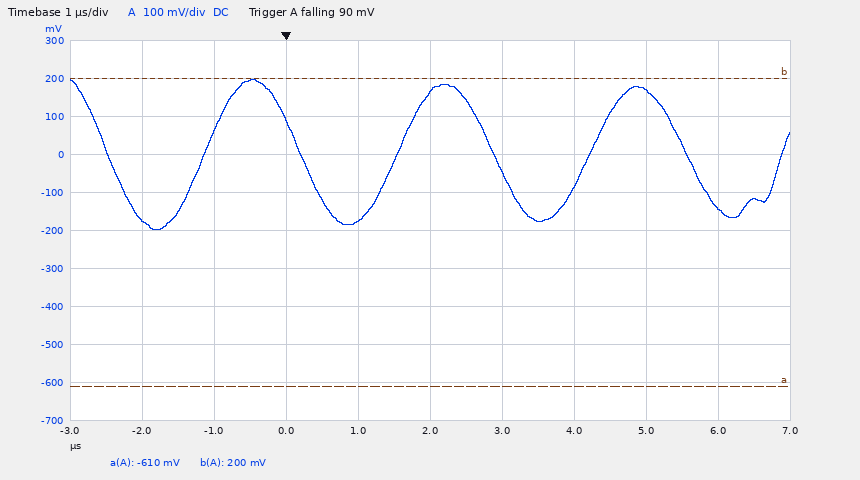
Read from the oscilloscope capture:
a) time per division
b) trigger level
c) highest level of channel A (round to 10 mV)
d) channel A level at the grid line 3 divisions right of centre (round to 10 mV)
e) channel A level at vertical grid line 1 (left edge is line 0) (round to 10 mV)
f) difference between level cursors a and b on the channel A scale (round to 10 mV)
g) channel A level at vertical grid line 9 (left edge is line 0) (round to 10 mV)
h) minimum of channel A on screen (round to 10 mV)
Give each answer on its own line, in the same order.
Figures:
1 µs
90 mV
200 mV
170 mV
-170 mV
810 mV
-140 mV
-200 mV
